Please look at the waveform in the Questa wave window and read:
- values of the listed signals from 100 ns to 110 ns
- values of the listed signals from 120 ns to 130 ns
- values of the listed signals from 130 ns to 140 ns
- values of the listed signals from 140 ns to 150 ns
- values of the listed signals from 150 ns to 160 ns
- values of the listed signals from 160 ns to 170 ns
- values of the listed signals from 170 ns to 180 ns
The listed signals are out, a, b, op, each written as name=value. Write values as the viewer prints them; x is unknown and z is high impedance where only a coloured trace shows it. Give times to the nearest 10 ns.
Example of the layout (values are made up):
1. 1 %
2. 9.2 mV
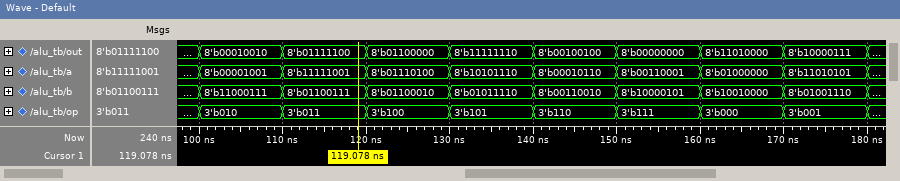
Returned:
1. out=8'b00010010, a=8'b00001001, b=8'b11000111, op=3'b010
2. out=8'b01100000, a=8'b01110100, b=8'b01100010, op=3'b100
3. out=8'b11111110, a=8'b10101110, b=8'b01011110, op=3'b101
4. out=8'b00100100, a=8'b00010110, b=8'b00110010, op=3'b110
5. out=8'b00000000, a=8'b00110001, b=8'b10000101, op=3'b111
6. out=8'b11010000, a=8'b01000000, b=8'b10010000, op=3'b000
7. out=8'b10000111, a=8'b11010101, b=8'b01001110, op=3'b001
